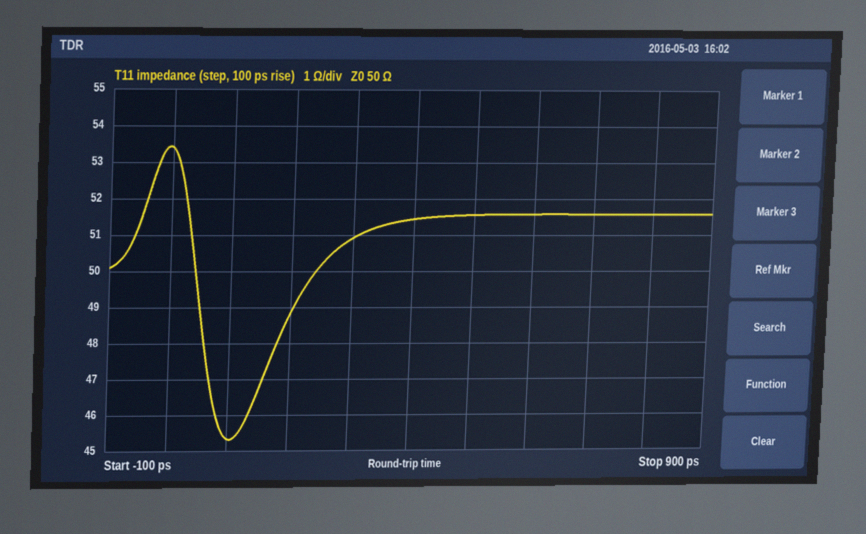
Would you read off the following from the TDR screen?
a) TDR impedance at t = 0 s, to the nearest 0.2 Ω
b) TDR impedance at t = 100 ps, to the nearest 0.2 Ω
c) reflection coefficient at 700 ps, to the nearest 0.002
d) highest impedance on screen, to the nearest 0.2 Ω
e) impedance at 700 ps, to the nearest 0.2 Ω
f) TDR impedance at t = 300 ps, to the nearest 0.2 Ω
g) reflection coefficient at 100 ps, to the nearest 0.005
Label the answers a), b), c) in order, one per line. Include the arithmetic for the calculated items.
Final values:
a) 53.4 Ω
b) 45.4 Ω
c) (51.6 − 50)/(51.6 + 50) ≈ +0.016
d) 53.4 Ω
e) 51.6 Ω
f) 51.0 Ω
g) (45.4 − 50)/(45.4 + 50) ≈ -0.0482, so -0.050 to the nearest 0.005
